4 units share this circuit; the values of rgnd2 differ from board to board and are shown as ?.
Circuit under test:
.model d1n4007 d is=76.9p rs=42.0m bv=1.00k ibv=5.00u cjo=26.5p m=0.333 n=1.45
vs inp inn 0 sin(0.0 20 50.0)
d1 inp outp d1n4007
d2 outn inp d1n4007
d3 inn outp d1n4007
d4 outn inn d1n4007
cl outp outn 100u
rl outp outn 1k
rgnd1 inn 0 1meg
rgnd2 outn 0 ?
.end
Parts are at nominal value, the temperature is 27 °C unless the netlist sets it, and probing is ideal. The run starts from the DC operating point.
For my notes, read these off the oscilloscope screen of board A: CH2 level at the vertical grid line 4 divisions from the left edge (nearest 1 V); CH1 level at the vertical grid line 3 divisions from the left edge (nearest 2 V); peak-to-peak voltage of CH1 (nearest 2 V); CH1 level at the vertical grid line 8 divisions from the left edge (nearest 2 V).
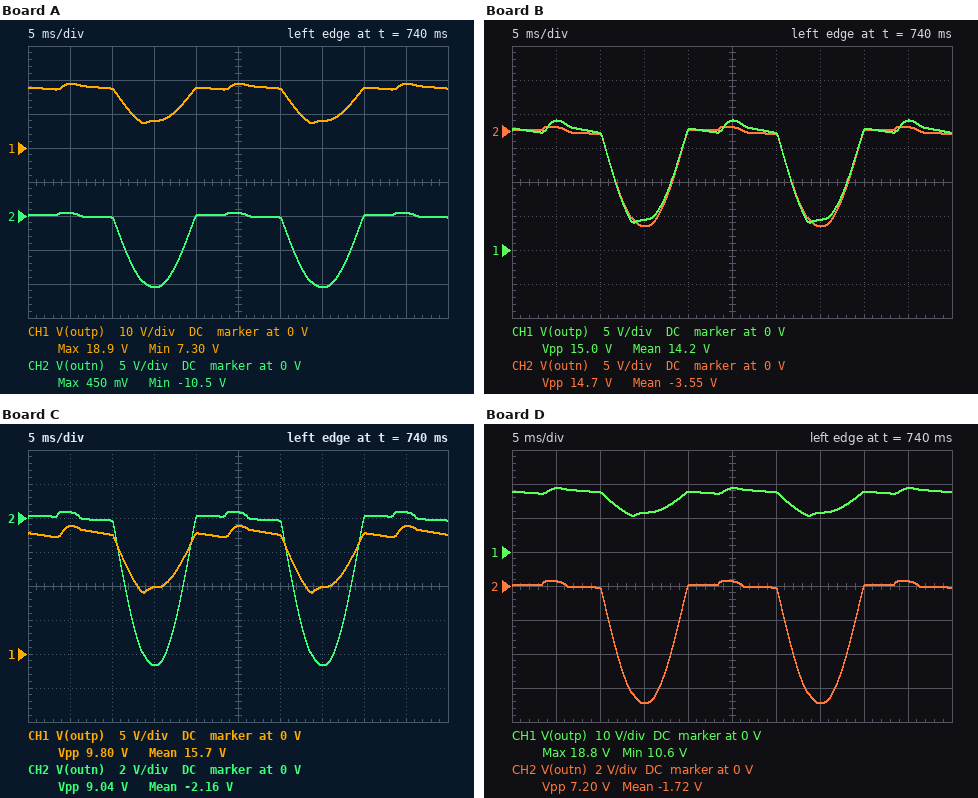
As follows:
0 V
8 V
12 V
18 V
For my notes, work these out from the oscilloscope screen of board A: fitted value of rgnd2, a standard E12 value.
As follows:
1.2 MΩ
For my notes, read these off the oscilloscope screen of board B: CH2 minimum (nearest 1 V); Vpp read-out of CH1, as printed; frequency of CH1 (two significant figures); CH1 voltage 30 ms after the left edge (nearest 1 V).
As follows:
-14 V
15.0 V
50 Hz
17 V
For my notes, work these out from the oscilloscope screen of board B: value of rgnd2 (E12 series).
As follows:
2.7 MΩ
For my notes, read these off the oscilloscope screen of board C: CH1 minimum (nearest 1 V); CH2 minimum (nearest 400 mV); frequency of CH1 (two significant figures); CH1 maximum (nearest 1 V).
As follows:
9 V
-8.8 V
50 Hz
19 V
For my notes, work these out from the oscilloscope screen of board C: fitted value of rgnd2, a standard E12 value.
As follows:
820 kΩ
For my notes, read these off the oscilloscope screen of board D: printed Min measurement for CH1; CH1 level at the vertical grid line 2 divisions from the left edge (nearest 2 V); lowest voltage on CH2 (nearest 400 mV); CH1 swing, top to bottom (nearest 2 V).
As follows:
10.6 V
18 V
-6.8 V
8 V
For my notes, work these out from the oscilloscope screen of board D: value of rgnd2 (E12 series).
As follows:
560 kΩ
